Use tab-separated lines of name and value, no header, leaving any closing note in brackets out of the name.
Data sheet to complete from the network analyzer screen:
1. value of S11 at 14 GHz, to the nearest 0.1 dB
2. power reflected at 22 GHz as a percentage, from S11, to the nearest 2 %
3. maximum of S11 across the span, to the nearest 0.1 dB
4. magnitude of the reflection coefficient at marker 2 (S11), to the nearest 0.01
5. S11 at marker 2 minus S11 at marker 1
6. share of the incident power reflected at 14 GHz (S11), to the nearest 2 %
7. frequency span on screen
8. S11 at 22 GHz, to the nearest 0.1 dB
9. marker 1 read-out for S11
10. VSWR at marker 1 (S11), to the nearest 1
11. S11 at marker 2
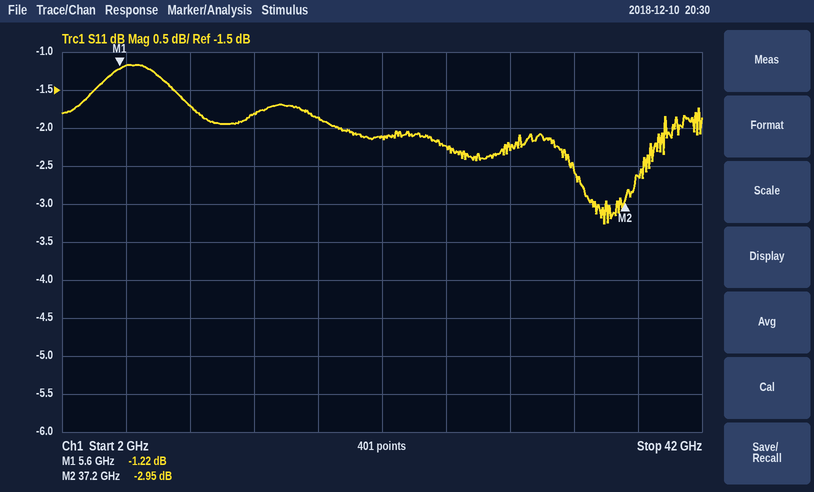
value of S11 at 14 GHz, to the nearest 0.1 dB	-1.8 dB
power reflected at 22 GHz as a percentage, from S11, to the nearest 2 %	62 %
maximum of S11 across the span, to the nearest 0.1 dB	-1.2 dB
magnitude of the reflection coefficient at marker 2 (S11), to the nearest 0.01	0.71
S11 at marker 2 minus S11 at marker 1	-1.73 dB
share of the incident power reflected at 14 GHz (S11), to the nearest 2 %	66 %
frequency span on screen	40 GHz
S11 at 22 GHz, to the nearest 0.1 dB	-2.1 dB
marker 1 read-out for S11	-1.22 dB
VSWR at marker 1 (S11), to the nearest 1	14
S11 at marker 2	-2.95 dB
